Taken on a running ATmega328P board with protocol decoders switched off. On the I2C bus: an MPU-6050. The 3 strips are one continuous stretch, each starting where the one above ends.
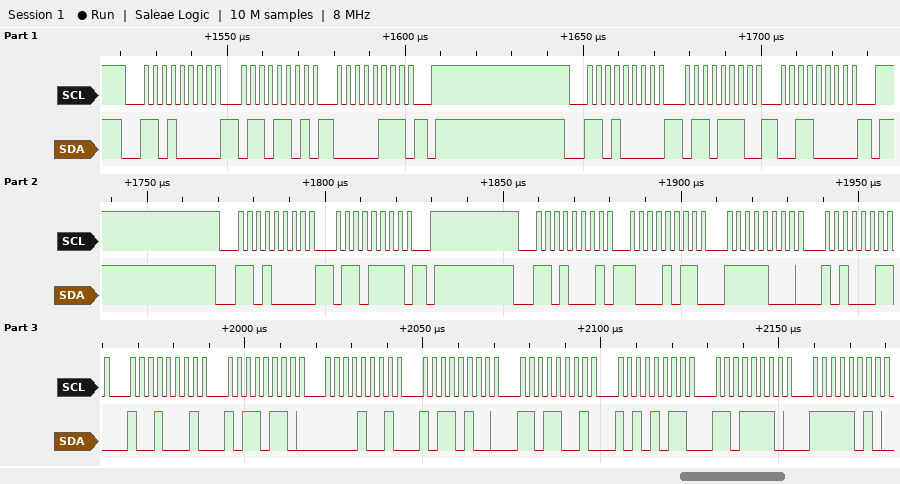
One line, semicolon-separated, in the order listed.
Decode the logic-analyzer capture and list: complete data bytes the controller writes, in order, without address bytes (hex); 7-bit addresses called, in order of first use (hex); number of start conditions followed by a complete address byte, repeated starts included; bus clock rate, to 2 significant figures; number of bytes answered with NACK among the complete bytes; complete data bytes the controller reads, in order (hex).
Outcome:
6D 07 6E 30 6F; 0x68; 4; 400 kHz; 0; 8B F8 A3 91 B6 09 B4 D9 AB DE FA
